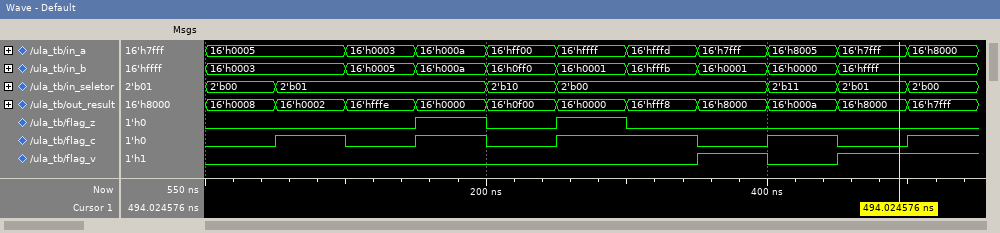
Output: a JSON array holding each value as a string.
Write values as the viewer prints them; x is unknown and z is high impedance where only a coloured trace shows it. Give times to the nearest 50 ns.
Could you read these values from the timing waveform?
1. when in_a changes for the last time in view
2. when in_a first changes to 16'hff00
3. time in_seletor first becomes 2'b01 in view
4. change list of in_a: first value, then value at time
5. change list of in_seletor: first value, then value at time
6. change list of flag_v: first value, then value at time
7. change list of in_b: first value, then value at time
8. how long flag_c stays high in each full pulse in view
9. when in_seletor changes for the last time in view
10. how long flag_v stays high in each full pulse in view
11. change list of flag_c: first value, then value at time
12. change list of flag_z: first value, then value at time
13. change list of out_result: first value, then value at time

["500 ns", "200 ns", "50 ns", "16'h0005, 16'h0003 at 100 ns, 16'h000a at 150 ns, 16'hff00 at 200 ns, 16'hffff at 250 ns, 16'hfffd at 300 ns, 16'h7fff at 350 ns, 16'h8005 at 400 ns, 16'h7fff at 450 ns, 16'h8000 at 500 ns", "2'b00, 2'b01 at 50 ns, 2'b10 at 200 ns, 2'b00 at 250 ns, 2'b11 at 400 ns, 2'b01 at 450 ns, 2'b00 at 500 ns", "0, 1 at 350 ns, 0 at 400 ns, 1 at 450 ns", "16'h0003, 16'h0005 at 100 ns, 16'h000a at 150 ns, 16'h0ff0 at 200 ns, 16'h0001 at 250 ns, 16'hfffb at 300 ns, 16'h0001 at 350 ns, 16'h0000 at 400 ns, 16'hffff at 450 ns", "50 ns, 50 ns, 100 ns, 50 ns", "500 ns", "50 ns", "0, 1 at 50 ns, 0 at 100 ns, 1 at 150 ns, 0 at 200 ns, 1 at 250 ns, 0 at 350 ns, 1 at 400 ns, 0 at 450 ns, 1 at 500 ns", "0, 1 at 150 ns, 0 at 200 ns, 1 at 250 ns, 0 at 300 ns", "16'h0008, 16'h0002 at 50 ns, 16'hfffe at 100 ns, 16'h0000 at 150 ns, 16'h0f00 at 200 ns, 16'h0000 at 250 ns, 16'hfff8 at 300 ns, 16'h8000 at 350 ns, 16'h000a at 400 ns, 16'h8000 at 450 ns, 16'h7fff at 500 ns"]
